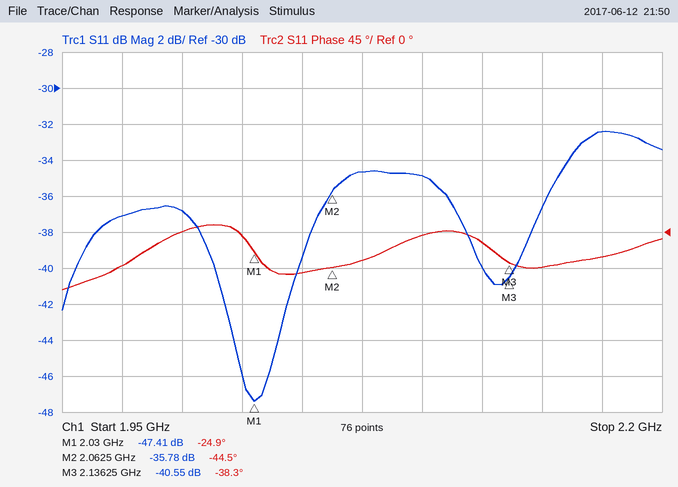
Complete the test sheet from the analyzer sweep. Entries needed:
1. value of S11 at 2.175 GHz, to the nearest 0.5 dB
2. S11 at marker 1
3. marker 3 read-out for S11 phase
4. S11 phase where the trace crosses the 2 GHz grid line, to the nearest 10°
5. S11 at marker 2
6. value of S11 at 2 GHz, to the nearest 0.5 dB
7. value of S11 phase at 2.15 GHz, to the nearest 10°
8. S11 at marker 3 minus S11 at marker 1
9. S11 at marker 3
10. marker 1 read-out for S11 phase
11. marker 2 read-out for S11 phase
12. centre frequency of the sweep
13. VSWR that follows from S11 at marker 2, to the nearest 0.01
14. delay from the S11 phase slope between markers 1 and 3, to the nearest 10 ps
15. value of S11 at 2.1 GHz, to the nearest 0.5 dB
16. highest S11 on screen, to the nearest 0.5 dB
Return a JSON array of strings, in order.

["-32.5 dB", "-47.41 dB", "-38.3°", "0°", "-35.78 dB", "-37.0 dB", "-40°", "6.86 dB", "-40.55 dB", "-24.9°", "-44.5°", "2.075 GHz", "1.03", "350 ps", "-35.0 dB", "-32.5 dB"]
